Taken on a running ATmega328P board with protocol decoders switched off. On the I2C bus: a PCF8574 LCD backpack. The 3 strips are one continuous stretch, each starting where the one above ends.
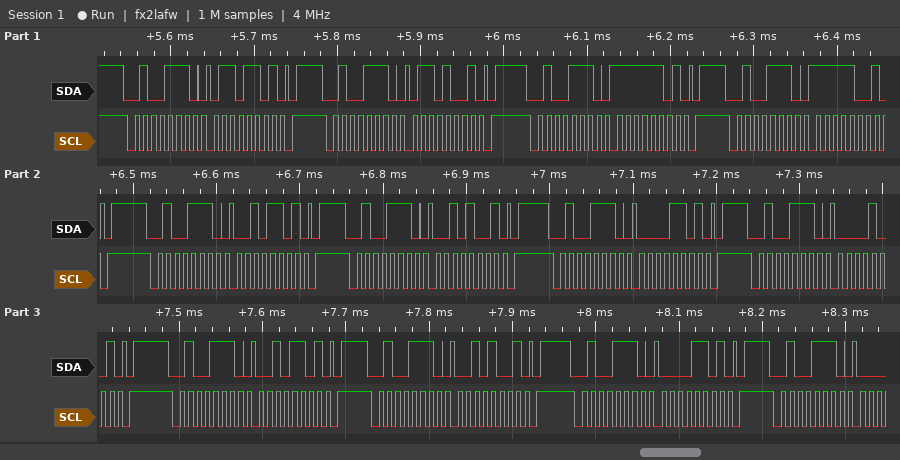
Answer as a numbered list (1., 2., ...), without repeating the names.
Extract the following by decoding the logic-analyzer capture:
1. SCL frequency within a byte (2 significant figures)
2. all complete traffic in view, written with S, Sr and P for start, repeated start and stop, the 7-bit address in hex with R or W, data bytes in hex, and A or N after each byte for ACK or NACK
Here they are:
1. 100 kHz
2. S 27W A 6D A P S 27W A 69 A P S 27W A FD A P S 27W A F9 A P S 27W A 2D A P S 27W A 29 A P S 27W A 0D A P S 27W A 09 A P S 27W A 2D A P S 27W A 29 A P S 27W A 0D A P S 27W A
